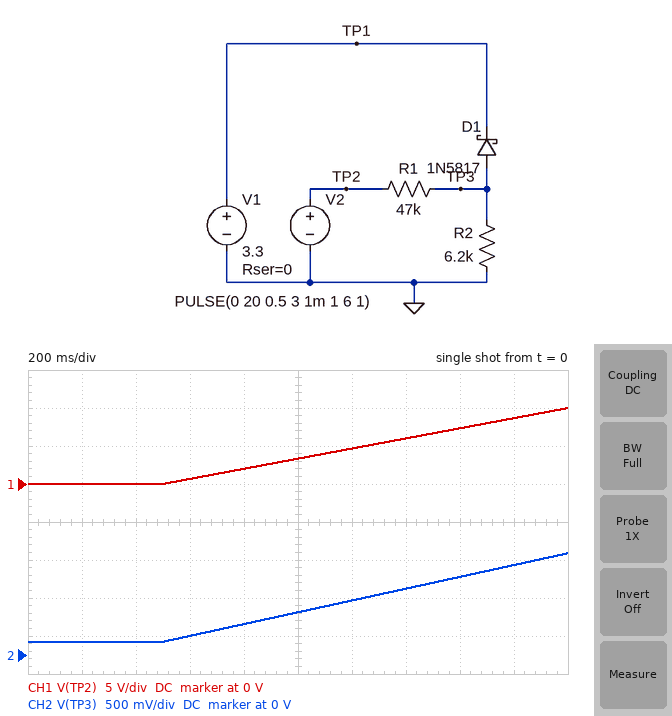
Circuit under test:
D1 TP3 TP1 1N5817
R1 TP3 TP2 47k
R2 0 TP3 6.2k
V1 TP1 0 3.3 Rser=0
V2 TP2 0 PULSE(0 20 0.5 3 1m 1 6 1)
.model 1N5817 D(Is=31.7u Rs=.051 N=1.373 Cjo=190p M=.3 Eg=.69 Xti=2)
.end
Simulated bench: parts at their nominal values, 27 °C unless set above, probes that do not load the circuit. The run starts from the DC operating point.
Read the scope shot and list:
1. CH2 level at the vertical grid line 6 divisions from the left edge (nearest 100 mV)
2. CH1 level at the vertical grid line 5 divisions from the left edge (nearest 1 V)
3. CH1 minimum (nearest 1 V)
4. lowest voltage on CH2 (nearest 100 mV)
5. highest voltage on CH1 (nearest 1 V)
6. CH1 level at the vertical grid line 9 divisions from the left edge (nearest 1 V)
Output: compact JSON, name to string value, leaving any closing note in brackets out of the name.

{"CH2 level at the vertical grid line 6 divisions from the left edge": "700 mV", "CH1 level at the vertical grid line 5 divisions from the left edge": "3 V", "CH1 minimum": "0 V", "lowest voltage on CH2": "200 mV", "highest voltage on CH1": "10 V", "CH1 level at the vertical grid line 9 divisions from the left edge": "9 V"}
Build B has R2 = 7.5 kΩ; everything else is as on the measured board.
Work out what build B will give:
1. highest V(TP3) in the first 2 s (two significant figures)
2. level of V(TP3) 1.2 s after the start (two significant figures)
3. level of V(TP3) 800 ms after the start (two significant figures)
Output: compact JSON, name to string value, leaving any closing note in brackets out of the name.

{"highest V(TP3) in the first 2 s": "1.6 V", "level of V(TP3) 1.2 s after the start": "850 mV", "level of V(TP3) 800 ms after the start": "480 mV"}
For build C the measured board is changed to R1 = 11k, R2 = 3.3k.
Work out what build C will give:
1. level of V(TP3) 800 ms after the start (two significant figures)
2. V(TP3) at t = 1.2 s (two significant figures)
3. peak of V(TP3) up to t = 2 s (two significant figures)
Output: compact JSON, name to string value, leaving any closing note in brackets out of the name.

{"level of V(TP3) 800 ms after the start": "540 mV", "V(TP3) at t = 1.2 s": "1.2 V", "peak of V(TP3) up to t = 2 s": "2.4 V"}
